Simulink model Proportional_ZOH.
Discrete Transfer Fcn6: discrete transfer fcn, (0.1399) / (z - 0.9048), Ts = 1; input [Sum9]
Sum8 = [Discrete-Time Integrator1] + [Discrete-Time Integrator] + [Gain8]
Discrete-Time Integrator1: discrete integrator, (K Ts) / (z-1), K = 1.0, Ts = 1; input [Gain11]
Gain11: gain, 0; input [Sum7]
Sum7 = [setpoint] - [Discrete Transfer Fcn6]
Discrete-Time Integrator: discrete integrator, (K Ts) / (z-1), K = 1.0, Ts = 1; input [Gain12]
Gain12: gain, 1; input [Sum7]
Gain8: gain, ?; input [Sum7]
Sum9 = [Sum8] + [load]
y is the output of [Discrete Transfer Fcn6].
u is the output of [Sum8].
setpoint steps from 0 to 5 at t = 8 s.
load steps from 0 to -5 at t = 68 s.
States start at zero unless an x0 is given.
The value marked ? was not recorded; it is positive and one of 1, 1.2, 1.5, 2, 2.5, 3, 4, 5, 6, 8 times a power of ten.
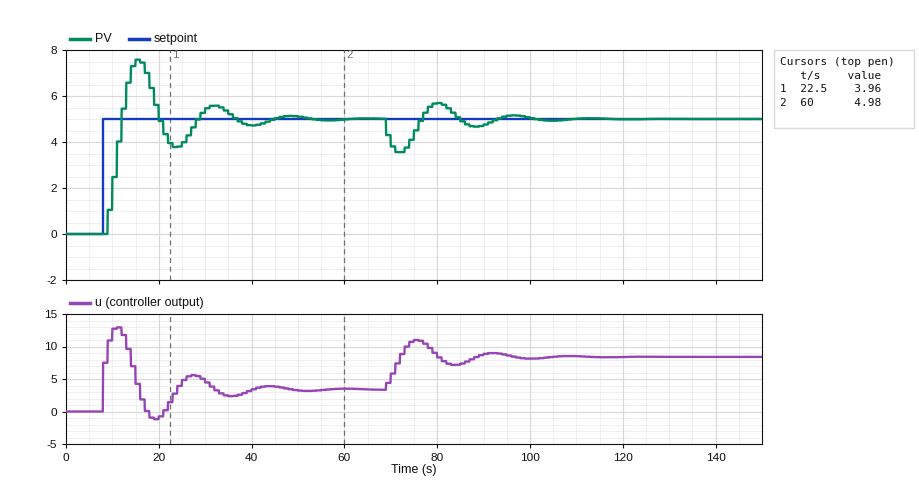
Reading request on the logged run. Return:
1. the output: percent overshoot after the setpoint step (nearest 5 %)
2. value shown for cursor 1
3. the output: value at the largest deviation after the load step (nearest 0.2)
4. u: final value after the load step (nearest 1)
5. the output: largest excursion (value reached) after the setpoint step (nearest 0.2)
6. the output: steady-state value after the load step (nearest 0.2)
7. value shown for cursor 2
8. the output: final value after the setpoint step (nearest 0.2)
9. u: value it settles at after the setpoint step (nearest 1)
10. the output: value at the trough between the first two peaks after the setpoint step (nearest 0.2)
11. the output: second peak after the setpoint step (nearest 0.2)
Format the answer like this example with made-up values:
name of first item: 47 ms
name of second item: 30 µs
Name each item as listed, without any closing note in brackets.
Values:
the output: percent overshoot after the setpoint step: 50 %
value shown for cursor 1: 3.96
the output: value at the largest deviation after the load step: 3.6
u: final value after the load step: 8
the output: largest excursion (value reached) after the setpoint step: 7.6
the output: steady-state value after the load step: 5.0
value shown for cursor 2: 4.98
the output: final value after the setpoint step: 5.0
u: value it settles at after the setpoint step: 3
the output: value at the trough between the first two peaks after the setpoint step: 3.8
the output: second peak after the setpoint step: 5.6
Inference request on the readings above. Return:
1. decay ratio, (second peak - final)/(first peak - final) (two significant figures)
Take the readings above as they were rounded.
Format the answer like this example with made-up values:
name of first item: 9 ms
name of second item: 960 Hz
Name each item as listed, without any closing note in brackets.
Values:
decay ratio, (second peak - final)/(first peak - final): 0.23
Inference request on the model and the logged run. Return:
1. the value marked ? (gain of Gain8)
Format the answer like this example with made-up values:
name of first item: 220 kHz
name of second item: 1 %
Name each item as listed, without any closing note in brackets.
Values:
the value marked ?: 1.5
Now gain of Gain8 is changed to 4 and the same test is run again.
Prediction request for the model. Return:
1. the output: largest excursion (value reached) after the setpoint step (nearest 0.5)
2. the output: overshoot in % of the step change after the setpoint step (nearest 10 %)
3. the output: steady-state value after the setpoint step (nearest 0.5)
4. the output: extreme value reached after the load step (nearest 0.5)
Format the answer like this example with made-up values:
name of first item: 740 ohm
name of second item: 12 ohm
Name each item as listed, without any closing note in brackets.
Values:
the output: largest excursion (value reached) after the setpoint step: 6.0
the output: overshoot in % of the step change after the setpoint step: 20 %
the output: steady-state value after the setpoint step: 5.0
the output: extreme value reached after the load step: 4.0
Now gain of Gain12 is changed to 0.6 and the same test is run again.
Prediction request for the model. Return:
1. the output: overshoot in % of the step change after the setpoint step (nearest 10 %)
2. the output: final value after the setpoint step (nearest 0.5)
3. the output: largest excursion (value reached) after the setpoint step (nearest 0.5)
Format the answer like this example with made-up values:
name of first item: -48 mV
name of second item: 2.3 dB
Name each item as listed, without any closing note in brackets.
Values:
the output: overshoot in % of the step change after the setpoint step: 30 %
the output: final value after the setpoint step: 5.0
the output: largest excursion (value reached) after the setpoint step: 6.5
